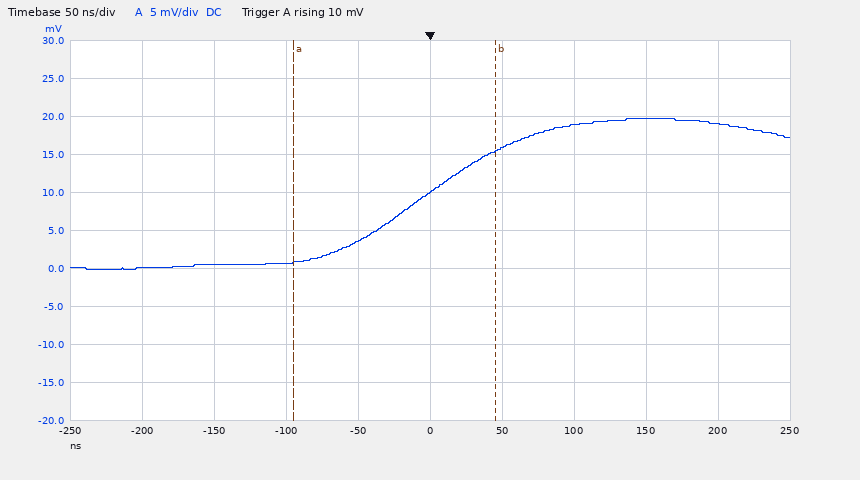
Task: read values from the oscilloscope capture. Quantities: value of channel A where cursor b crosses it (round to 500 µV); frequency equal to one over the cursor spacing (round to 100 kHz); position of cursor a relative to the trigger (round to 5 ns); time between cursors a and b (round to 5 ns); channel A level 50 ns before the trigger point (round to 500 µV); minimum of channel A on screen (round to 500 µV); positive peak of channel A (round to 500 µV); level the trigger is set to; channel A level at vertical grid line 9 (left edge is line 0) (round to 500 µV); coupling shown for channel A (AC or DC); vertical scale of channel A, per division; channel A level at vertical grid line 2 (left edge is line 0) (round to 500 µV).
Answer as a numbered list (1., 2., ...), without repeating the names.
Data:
1. 15.5 mV
2. 7.1 MHz
3. -95 ns
4. 140 ns
5. 3.5 mV
6. 0.0 mV
7. 19.5 mV
8. 10 mV
9. 19.0 mV
10. DC
11. 5 mV
12. 500 µV
